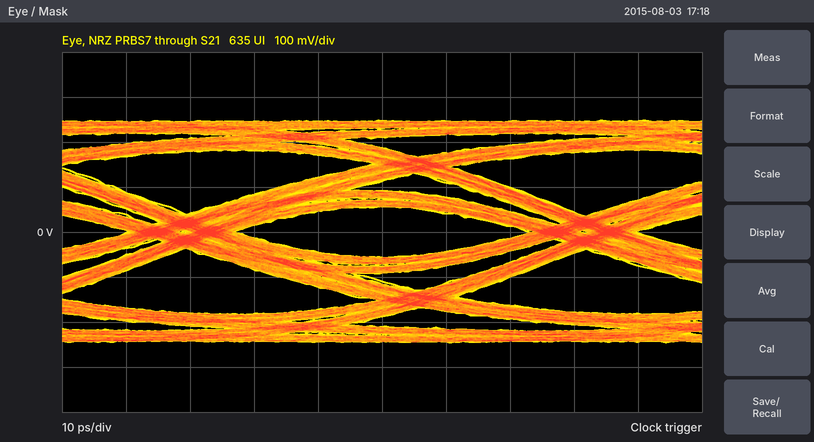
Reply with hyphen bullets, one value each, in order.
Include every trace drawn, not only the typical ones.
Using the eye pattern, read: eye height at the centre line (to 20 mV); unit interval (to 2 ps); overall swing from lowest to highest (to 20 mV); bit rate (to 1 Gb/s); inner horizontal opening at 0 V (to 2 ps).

- 120 mV
- 62 ps
- 500 mV
- 16 Gb/s
- 46 ps
